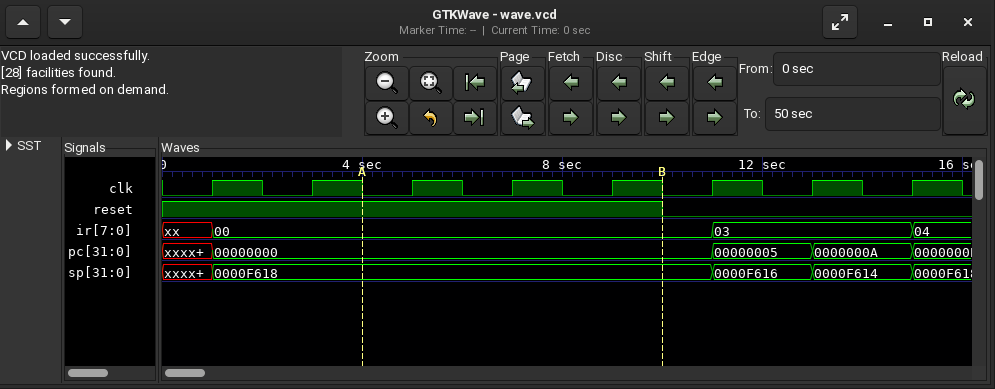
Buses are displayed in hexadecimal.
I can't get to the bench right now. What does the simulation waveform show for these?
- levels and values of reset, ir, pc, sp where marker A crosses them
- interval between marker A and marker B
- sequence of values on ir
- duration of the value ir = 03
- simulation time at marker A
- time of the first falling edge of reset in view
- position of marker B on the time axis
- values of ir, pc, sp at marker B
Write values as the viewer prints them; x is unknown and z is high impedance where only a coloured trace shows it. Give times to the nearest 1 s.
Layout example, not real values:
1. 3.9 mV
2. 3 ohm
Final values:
1. reset=1, ir=00, pc=00000000, sp=0000F618
2. 6 s
3. xx, 00, 03, 04
4. 4 s
5. 4 s
6. 10 s
7. 10 s
8. ir=00, pc=00000000, sp=0000F618
